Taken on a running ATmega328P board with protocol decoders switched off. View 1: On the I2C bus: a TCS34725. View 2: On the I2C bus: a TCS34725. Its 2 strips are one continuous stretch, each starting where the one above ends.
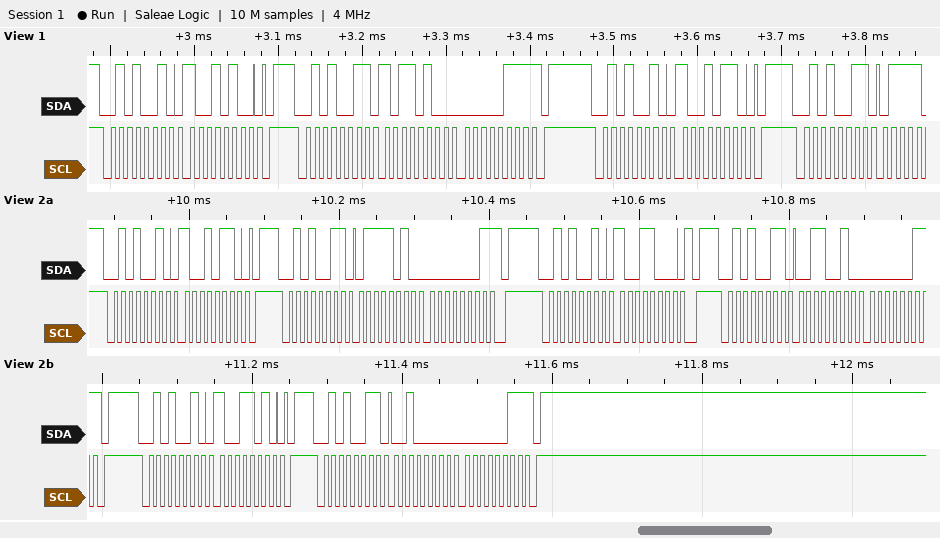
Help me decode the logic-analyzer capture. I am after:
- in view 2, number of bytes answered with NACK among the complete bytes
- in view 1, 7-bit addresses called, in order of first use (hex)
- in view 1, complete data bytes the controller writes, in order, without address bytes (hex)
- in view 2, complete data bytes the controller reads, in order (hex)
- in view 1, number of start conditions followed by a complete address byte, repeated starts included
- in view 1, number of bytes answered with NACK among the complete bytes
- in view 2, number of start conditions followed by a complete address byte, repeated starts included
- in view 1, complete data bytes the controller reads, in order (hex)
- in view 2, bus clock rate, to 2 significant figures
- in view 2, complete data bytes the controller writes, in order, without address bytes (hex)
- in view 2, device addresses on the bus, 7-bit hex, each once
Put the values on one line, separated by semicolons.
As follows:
3; 0x29; 94 96; 7A 01 32 03 20 03; 4; 1; 6; B4 07; 100 kHz; 96 98 9A; 0x29
